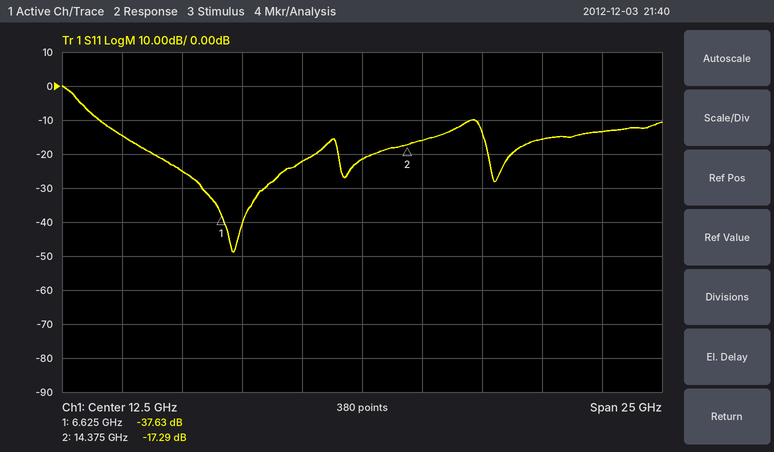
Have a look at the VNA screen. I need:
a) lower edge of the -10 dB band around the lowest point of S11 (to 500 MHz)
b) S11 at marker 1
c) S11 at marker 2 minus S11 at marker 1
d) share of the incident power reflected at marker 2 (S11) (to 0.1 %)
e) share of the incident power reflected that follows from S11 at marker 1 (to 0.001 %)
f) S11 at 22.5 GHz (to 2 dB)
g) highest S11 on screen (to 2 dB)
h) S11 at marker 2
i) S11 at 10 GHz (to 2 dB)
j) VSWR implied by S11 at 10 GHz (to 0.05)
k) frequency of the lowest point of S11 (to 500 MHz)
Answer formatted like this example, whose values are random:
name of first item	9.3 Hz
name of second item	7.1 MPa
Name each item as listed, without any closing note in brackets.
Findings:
lower edge of the -10 dB band around the lowest point of S11	1.5 GHz
S11 at marker 1	-37.63 dB
S11 at marker 2 minus S11 at marker 1	20.34 dB
share of the incident power reflected at marker 2 (S11)	1.9 %
share of the incident power reflected that follows from S11 at marker 1	0.017 %
S11 at 22.5 GHz	-14 dB
highest S11 on screen	0 dB
S11 at marker 2	-17.29 dB
S11 at 10 GHz	-22 dB
VSWR implied by S11 at 10 GHz	1.15
frequency of the lowest point of S11	7.0 GHz
